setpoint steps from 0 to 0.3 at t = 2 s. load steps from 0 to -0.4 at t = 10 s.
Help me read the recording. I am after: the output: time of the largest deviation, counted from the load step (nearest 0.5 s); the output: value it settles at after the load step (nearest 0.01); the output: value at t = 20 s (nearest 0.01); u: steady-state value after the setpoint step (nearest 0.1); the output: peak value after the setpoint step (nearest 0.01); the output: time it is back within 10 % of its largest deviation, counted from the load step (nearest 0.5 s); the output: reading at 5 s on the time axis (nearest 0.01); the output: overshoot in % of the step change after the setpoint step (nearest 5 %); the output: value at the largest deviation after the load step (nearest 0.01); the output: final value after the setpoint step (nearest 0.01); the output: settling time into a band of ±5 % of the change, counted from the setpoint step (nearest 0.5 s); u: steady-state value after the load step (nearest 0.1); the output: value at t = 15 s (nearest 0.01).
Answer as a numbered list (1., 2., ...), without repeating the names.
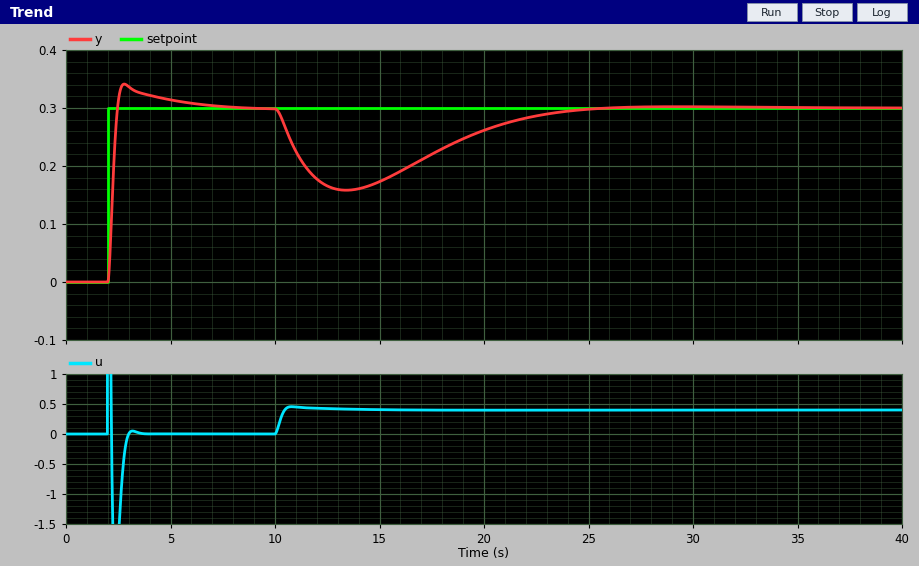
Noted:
1. 3.5 s
2. 0.30
3. 0.26
4. 0.0
5. 0.34
6. 12.5 s
7. 0.31
8. 15 %
9. 0.16
10. 0.30
11. 3.0 s
12. 0.4
13. 0.17
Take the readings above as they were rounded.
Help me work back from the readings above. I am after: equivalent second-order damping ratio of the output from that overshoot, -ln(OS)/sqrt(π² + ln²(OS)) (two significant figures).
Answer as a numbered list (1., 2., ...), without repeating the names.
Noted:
1. 0.52
